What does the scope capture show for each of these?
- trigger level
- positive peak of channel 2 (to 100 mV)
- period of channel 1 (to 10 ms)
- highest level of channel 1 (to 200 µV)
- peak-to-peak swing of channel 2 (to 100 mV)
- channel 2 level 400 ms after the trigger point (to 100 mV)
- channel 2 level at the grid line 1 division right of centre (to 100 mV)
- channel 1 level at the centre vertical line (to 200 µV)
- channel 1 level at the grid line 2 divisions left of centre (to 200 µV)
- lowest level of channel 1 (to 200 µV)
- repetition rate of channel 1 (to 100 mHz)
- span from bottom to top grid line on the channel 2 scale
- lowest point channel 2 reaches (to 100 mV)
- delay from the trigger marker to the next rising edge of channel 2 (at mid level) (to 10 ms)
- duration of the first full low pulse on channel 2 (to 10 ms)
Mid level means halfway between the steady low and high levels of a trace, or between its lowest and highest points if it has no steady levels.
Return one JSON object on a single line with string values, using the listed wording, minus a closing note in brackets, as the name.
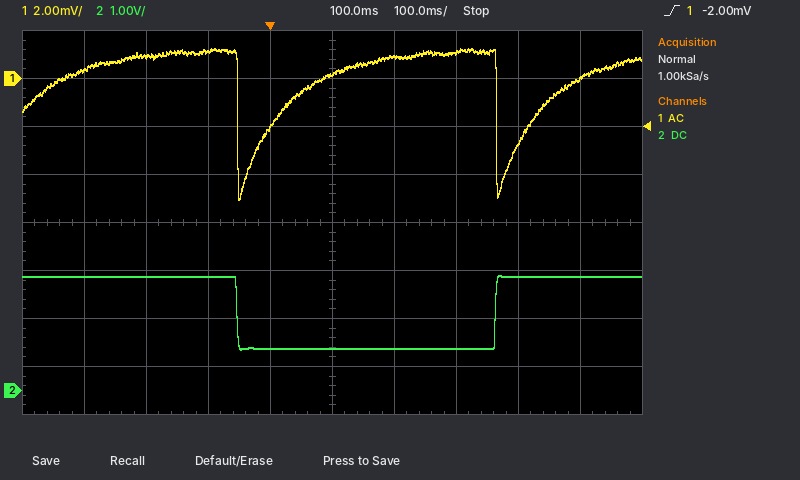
{"trigger level": "-2.00 mV", "positive peak of channel 2": "2.4 V", "period of channel 1": "420 ms", "highest level of channel 1": "1.2 mV", "peak-to-peak swing of channel 2": "1.5 V", "channel 2 level 400 ms after the trigger point": "2.4 V", "channel 2 level at the grid line 1 division right of centre": "900 mV", "channel 1 level at the centre vertical line": "200 µV", "channel 1 level at the grid line 2 divisions left of centre": "1.2 mV", "lowest level of channel 1": "-5.0 mV", "repetition rate of channel 1": "2.4 Hz", "span from bottom to top grid line on the channel 2 scale": "8 V", "lowest point channel 2 reaches": "900 mV", "delay from the trigger marker to the next rising edge of channel 2 (at mid level)": "360 ms", "duration of the first full low pulse on channel 2": "420 ms"}
